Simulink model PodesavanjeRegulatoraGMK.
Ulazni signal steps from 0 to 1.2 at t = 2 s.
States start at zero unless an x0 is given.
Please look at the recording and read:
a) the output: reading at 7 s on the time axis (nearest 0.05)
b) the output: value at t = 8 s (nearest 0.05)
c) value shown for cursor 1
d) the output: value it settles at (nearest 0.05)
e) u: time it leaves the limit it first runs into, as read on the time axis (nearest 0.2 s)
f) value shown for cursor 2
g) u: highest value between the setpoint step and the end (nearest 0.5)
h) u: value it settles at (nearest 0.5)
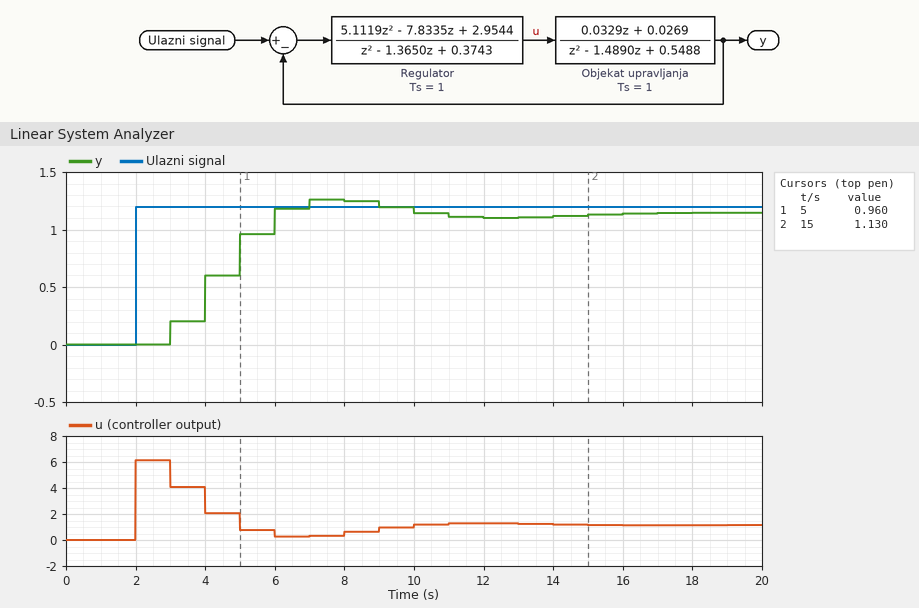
1.25
1.25
0.960
1.15
3.0 s
1.130
6.0
1.0
